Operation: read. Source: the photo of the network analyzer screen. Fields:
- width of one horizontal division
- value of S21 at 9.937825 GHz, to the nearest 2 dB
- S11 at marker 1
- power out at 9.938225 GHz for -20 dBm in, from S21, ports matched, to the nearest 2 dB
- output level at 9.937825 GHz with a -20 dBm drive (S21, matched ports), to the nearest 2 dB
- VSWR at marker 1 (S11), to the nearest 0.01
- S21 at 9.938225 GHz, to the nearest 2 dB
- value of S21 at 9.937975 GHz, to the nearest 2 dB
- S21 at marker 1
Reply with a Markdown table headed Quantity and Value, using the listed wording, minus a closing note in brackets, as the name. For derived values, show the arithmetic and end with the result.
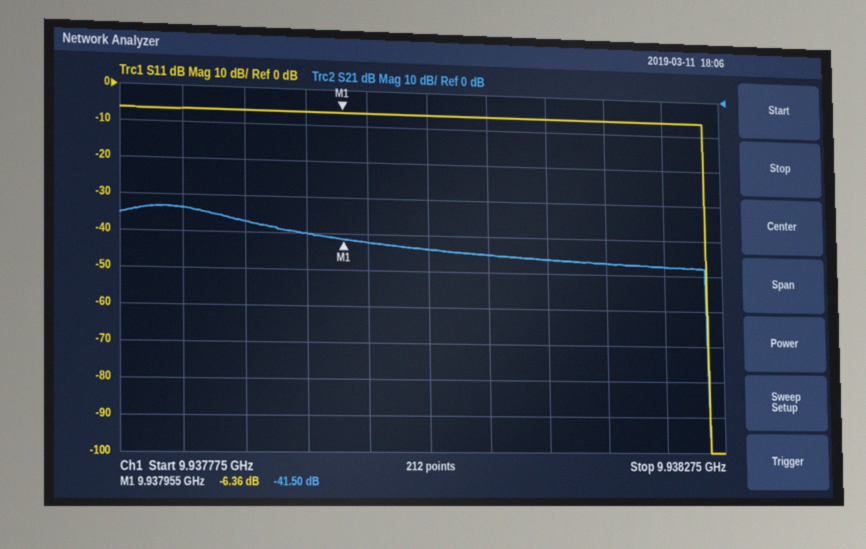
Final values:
| Quantity | Value |
|---|---|
| width of one horizontal division | 50 kHz |
| value of S21 at 9.937825 GHz, to the nearest 2 dB | -34 dB |
| S11 at marker 1 | -6.36 dB |
| power out at 9.938225 GHz for -20 dBm in, from S21, ports matched, to the nearest 2 dB | -20 dBm + (-48 dB) = -68 dBm |
| output level at 9.937825 GHz with a -20 dBm drive (S21, matched ports), to the nearest 2 dB | -20 dBm + (-34 dB) = -54 dBm |
| VSWR at marker 1 (S11), to the nearest 0.01 | (1 + 0.4808)/(1 − 0.4808) ≈ 2.85 |
| S21 at 9.938225 GHz, to the nearest 2 dB | -48 dB |
| value of S21 at 9.937975 GHz, to the nearest 2 dB | -42 dB |
| S21 at marker 1 | -41.50 dB |
